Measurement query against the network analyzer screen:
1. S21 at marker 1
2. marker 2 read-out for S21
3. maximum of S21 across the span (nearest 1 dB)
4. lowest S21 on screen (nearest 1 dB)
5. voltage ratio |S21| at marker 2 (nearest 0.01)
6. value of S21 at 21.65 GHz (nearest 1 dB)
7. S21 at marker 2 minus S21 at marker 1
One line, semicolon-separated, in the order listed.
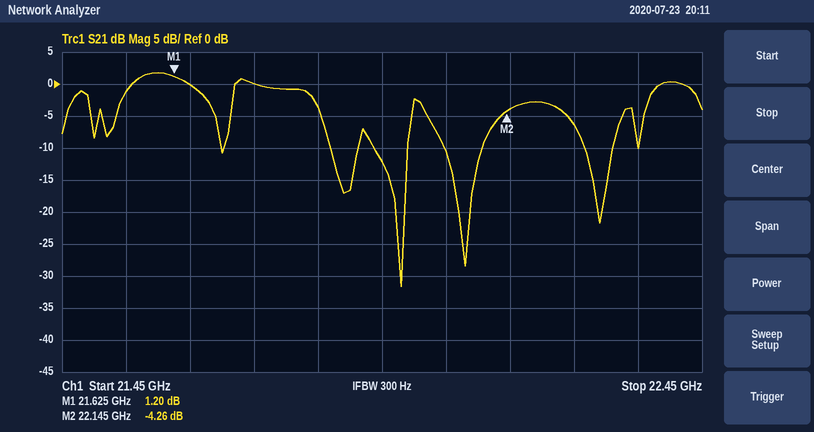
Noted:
1.20 dB; -4.26 dB; 2 dB; -32 dB; 0.61; 0 dB; -5.46 dB
